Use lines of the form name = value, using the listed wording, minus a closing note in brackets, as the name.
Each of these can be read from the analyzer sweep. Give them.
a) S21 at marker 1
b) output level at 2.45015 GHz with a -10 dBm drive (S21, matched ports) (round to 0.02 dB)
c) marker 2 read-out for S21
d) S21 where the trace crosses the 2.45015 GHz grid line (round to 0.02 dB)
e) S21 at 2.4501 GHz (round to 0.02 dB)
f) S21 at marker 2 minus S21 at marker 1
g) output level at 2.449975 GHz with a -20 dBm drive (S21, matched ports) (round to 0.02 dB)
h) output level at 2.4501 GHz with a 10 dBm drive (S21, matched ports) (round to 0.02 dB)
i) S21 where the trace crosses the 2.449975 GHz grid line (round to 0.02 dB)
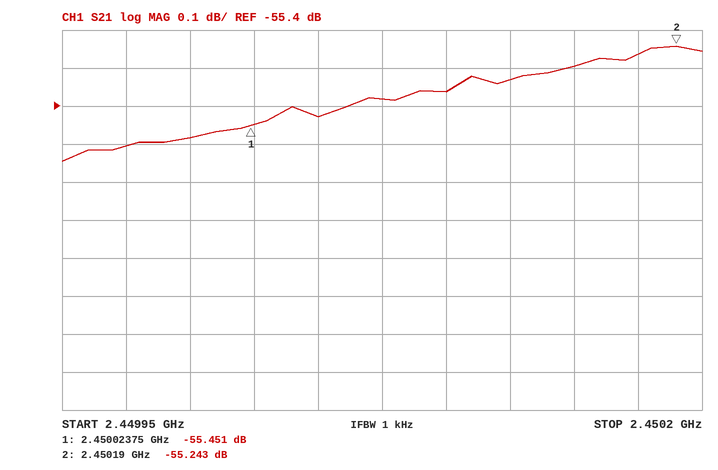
S21 at marker 1 = -55.451 dB
output level at 2.45015 GHz with a -10 dBm drive (S21, matched ports) = -65.30 dBm
marker 2 read-out for S21 = -55.243 dB
S21 where the trace crosses the 2.45015 GHz grid line = -55.30 dB
S21 at 2.4501 GHz = -55.36 dB
S21 at marker 2 minus S21 at marker 1 = 0.208 dB
output level at 2.449975 GHz with a -20 dBm drive (S21, matched ports) = -75.50 dBm
output level at 2.4501 GHz with a 10 dBm drive (S21, matched ports) = -45.36 dBm
S21 where the trace crosses the 2.449975 GHz grid line = -55.50 dB
